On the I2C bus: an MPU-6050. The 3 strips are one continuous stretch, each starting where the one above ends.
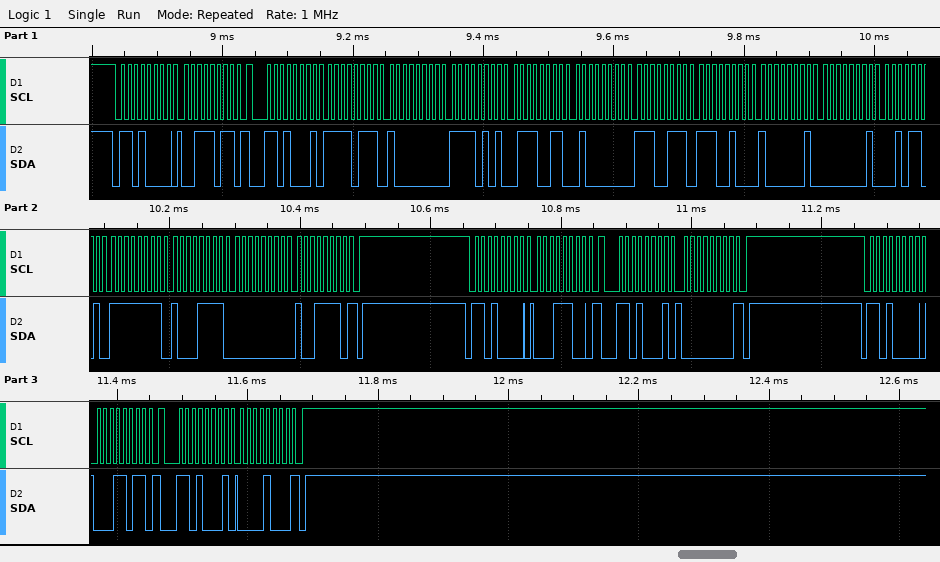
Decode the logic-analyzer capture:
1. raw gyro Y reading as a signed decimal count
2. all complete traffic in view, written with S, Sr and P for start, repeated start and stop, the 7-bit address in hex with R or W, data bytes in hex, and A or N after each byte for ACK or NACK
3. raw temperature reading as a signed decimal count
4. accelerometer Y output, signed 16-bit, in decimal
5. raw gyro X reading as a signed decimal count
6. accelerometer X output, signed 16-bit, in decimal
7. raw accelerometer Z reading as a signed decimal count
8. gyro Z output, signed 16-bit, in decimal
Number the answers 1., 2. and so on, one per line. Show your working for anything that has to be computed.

1. 0xFF8F = -113
2. S 68W A 3B A Sr 68R A F7 A 80 A F5 A 73 A 40 A E7 A E4 A 81 A 01 A 2D A FF A 8F A 00 A 9E N P S 68W A 1C A Sr 68R A 00 N P S 68W A 1B A Sr 68R A 08 N P
3. 0xE481 = -7039
4. 0xF573 = -2701
5. 0x012D = 301
6. 0xF780 = -2176
7. 0x40E7 = 16615
8. 0x009E = 158
